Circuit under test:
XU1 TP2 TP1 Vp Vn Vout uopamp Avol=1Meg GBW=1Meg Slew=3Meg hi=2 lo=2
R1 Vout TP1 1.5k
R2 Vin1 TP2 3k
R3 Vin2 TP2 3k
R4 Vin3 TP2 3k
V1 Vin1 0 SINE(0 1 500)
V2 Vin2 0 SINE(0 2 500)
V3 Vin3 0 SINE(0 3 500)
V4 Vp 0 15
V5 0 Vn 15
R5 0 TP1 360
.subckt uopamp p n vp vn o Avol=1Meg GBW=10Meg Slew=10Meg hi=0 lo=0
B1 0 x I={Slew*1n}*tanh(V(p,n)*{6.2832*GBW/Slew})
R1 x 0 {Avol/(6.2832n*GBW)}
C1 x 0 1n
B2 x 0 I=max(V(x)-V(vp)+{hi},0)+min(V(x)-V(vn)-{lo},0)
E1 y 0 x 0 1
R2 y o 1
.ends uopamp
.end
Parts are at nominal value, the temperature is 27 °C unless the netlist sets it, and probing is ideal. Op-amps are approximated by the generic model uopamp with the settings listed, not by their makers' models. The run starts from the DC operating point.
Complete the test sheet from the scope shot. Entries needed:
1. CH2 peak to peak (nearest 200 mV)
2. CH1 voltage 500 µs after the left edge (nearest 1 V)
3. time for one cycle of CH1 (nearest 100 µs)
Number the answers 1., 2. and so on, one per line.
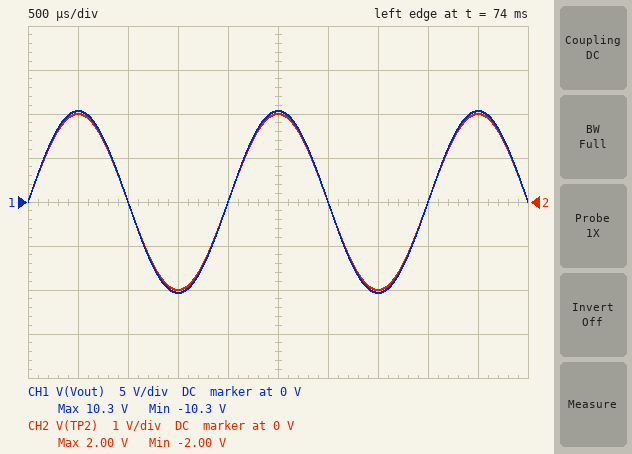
1. 4.0 V
2. 10 V
3. 2.0 ms
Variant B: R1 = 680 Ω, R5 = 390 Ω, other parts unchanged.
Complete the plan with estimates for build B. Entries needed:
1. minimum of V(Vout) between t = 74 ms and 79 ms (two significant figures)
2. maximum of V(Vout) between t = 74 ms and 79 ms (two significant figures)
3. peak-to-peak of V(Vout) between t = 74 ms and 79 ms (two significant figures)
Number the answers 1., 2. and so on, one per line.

1. -5.5 V
2. 5.5 V
3. 11 V
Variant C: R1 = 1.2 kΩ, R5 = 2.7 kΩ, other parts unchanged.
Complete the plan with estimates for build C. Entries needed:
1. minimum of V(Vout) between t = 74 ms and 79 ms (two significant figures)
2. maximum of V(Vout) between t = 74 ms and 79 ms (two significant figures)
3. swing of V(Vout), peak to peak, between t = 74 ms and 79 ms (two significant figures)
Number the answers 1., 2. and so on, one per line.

1. -2.9 V
2. 2.9 V
3. 5.8 V
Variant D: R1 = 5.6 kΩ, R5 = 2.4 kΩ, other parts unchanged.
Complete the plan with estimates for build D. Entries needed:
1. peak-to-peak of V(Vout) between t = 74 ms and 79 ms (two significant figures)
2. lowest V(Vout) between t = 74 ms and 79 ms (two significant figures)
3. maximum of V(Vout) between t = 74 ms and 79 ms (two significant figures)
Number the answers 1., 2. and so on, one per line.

1. 13 V
2. -6.7 V
3. 6.7 V
